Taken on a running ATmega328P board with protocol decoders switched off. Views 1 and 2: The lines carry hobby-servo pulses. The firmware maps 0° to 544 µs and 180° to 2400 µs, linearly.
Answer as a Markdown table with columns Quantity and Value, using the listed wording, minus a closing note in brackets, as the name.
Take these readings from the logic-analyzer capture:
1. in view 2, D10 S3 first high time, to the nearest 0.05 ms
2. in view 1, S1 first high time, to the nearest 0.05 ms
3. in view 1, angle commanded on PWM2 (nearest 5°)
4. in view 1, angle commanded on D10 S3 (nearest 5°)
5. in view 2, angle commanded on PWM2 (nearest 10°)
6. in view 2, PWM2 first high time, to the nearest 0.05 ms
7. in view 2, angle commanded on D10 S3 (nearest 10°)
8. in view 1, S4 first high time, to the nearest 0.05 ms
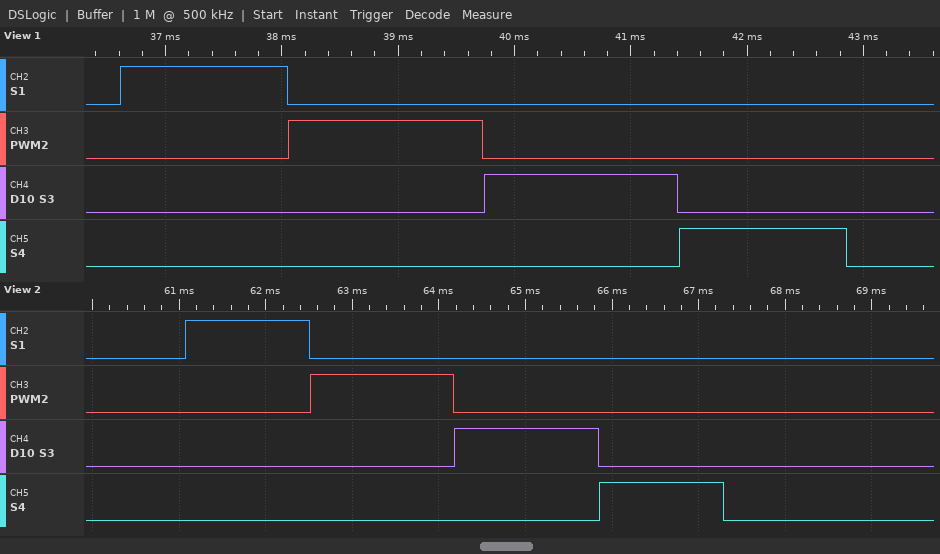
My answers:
| Quantity | Value |
|---|---|
| in view 2, D10 S3 first high time, to the nearest 0.05 ms | 1.65 ms |
| in view 1, S1 first high time, to the nearest 0.05 ms | 1.45 ms |
| in view 1, angle commanded on PWM2 | 110° |
| in view 1, angle commanded on D10 S3 | 110° |
| in view 2, angle commanded on PWM2 | 110° |
| in view 2, PWM2 first high time, to the nearest 0.05 ms | 1.65 ms |
| in view 2, angle commanded on D10 S3 | 110° |
| in view 1, S4 first high time, to the nearest 0.05 ms | 1.45 ms |
